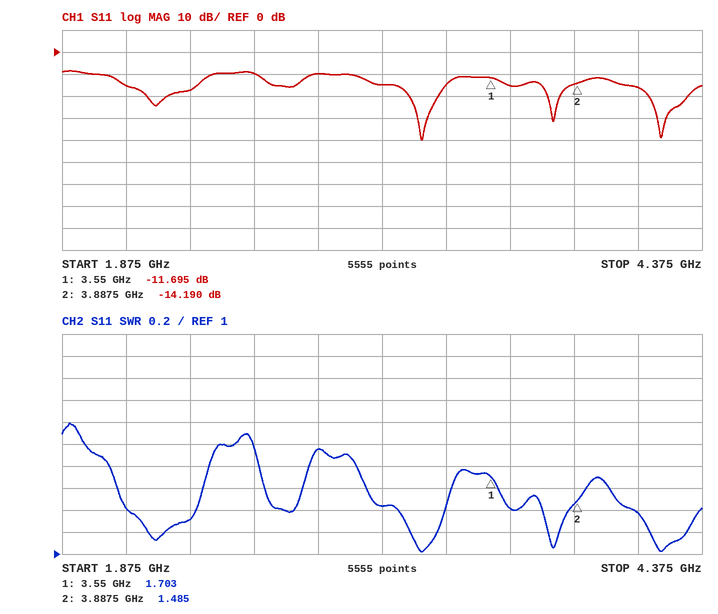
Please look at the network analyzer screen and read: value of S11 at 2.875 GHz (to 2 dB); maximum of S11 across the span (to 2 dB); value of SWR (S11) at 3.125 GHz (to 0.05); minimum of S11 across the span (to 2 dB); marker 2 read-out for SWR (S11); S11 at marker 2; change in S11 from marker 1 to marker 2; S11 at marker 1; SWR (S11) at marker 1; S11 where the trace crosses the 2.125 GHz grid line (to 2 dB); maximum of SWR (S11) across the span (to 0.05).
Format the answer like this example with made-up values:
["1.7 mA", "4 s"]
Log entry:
["-10 dB", "-8 dB", "1.45", "-40 dB", "1.485", "-14.190 dB", "-2.495 dB", "-11.695 dB", "1.703", "-16 dB", "2.20"]
